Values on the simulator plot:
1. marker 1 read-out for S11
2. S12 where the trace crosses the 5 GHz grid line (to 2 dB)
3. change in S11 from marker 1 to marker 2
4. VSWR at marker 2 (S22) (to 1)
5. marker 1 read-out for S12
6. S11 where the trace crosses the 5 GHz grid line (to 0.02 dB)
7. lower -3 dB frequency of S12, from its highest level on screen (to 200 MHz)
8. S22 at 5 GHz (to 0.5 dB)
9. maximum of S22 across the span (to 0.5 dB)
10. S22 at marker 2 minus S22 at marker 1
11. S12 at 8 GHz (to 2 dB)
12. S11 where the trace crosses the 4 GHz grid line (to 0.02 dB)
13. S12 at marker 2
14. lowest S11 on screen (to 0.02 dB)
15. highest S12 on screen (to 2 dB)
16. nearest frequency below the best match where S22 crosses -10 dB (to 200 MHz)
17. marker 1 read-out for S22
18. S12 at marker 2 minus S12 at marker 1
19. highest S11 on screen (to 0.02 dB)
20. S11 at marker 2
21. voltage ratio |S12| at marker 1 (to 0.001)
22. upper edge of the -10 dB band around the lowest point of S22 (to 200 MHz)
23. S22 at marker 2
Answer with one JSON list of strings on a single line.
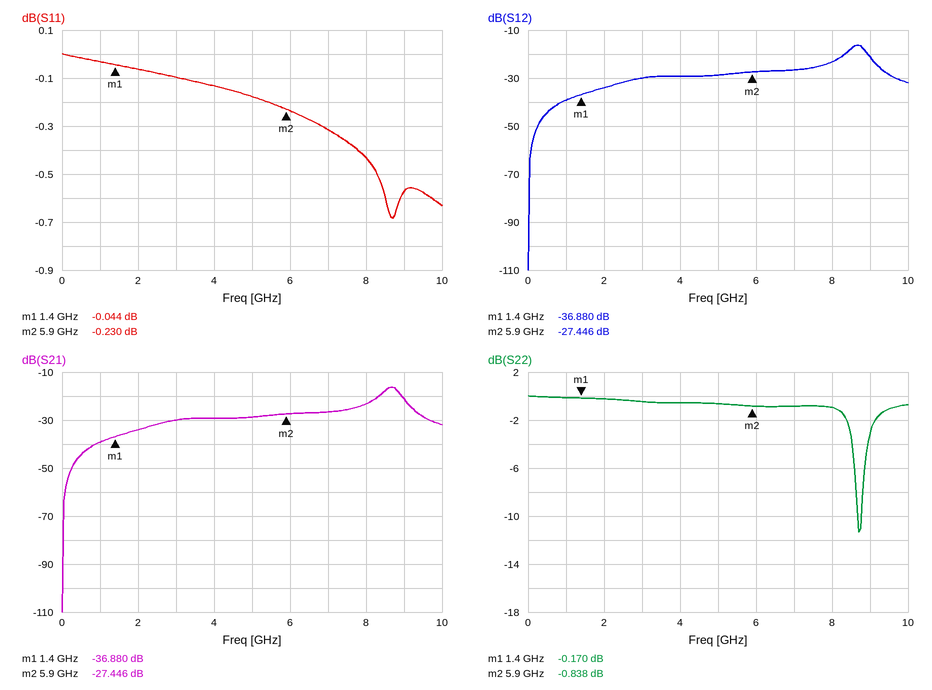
["-0.044 dB", "-28 dB", "-0.186 dB", "21", "-36.880 dB", "-0.18 dB", "8.4 GHz", "-0.5 dB", "0.0 dB", "-0.668 dB", "-24 dB", "-0.14 dB", "-27.446 dB", "-0.68 dB", "-16 dB", "8.6 GHz", "-0.170 dB", "9.434 dB", "0.00 dB", "-0.230 dB", "0.014", "8.8 GHz", "-0.838 dB"]
